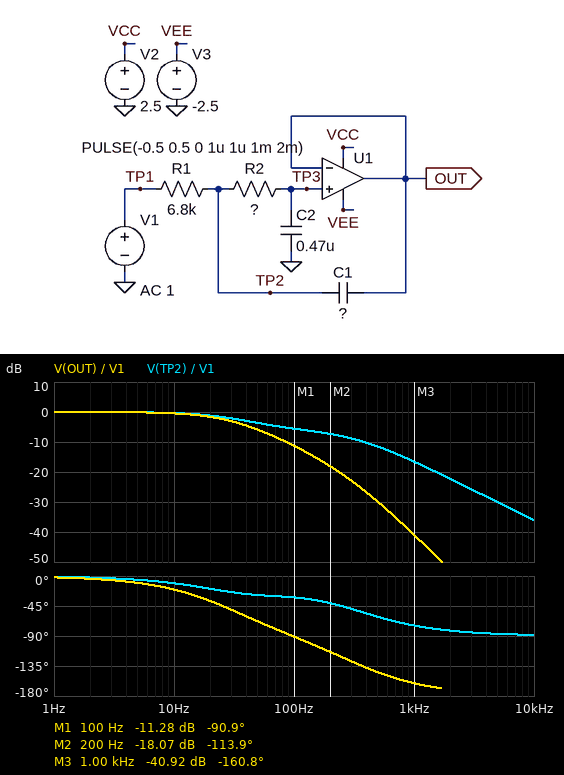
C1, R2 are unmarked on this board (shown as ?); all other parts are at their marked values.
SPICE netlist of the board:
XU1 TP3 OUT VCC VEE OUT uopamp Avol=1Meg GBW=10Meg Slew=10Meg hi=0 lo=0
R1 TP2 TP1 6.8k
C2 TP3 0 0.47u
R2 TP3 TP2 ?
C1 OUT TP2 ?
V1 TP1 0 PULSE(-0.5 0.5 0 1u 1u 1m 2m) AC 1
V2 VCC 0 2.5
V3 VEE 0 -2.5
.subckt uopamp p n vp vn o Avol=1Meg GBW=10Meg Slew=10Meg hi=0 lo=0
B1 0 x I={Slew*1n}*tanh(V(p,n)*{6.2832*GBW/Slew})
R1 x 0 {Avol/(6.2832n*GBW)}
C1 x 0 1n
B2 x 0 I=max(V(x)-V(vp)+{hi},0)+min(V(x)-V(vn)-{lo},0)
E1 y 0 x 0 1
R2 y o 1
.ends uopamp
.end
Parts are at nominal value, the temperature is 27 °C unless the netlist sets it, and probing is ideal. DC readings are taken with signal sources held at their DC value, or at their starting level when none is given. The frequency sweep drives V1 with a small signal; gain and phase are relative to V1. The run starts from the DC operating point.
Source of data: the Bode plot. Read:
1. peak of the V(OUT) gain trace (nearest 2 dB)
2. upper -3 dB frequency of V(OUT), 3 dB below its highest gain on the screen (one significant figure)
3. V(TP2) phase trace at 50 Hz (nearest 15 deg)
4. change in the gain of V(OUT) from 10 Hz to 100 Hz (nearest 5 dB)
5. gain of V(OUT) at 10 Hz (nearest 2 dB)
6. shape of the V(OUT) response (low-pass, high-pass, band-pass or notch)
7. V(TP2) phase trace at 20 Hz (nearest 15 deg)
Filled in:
0 dB
30 Hz
-30 deg
-10 dB
0 dB
low-pass
-15 deg
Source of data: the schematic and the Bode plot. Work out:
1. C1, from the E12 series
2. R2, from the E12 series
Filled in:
150 nF
5.6 kΩ
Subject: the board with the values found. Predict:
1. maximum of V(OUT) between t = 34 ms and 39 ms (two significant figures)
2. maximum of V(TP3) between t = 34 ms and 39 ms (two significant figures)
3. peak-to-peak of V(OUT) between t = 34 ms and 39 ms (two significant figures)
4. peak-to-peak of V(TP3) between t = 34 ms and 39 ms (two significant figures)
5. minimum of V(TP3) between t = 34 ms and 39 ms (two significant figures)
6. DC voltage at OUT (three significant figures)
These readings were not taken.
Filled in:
20 mV
20 mV
41 mV
41 mV
-21 mV
-500 mV
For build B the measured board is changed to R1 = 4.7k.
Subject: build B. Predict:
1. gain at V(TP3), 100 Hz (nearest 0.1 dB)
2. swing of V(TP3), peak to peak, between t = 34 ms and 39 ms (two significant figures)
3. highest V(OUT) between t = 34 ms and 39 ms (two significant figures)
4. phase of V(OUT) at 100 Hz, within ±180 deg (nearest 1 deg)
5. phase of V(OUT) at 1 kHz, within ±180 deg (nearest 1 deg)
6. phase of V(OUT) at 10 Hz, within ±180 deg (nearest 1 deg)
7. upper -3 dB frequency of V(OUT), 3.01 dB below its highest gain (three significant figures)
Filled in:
-9.7 dB
56 mV
28 mV
-85 deg
-157 deg
-17 deg
35.7 Hz
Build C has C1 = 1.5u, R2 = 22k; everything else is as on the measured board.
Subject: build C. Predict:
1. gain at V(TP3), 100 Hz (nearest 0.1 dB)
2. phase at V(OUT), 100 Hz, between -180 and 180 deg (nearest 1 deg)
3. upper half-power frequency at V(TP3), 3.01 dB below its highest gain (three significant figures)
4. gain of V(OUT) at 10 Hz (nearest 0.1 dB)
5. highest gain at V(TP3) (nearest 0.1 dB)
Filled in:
-32.4 dB
-168 deg
16.4 Hz
-0.3 dB
0.1 dB
